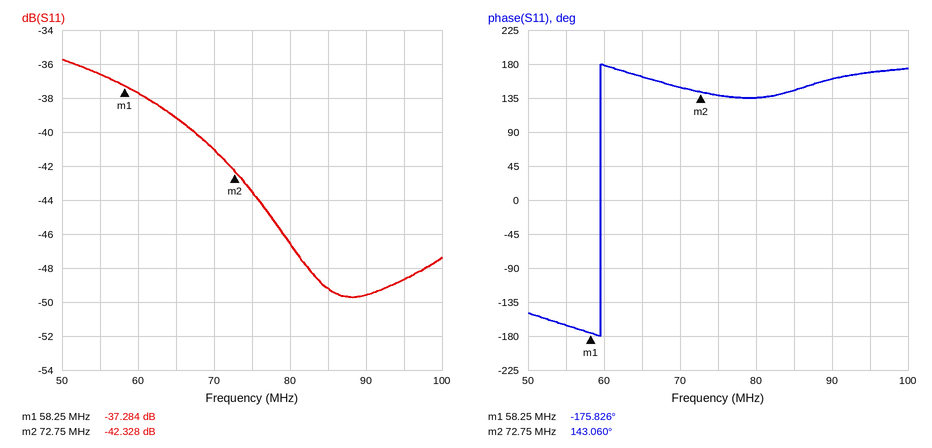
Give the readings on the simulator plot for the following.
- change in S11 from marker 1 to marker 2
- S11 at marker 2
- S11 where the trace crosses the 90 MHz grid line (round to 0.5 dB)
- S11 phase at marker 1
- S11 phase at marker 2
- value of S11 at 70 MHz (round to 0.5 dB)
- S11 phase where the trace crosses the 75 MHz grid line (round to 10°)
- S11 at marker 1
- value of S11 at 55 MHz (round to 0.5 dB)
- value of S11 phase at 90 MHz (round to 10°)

-5.044 dB
-42.328 dB
-49.5 dB
-175.826°
143.060°
-41.0 dB
140°
-37.284 dB
-36.5 dB
160°
